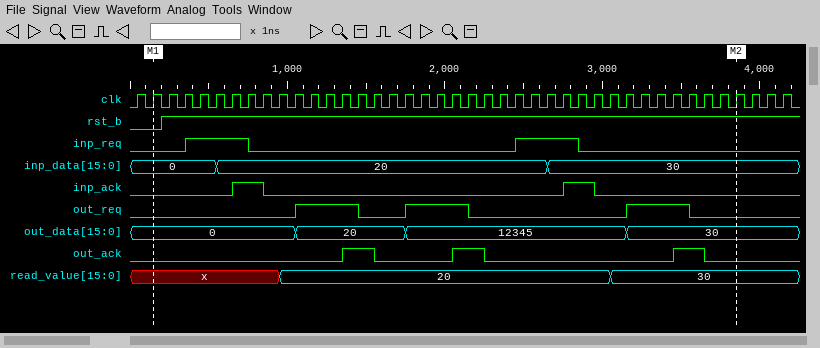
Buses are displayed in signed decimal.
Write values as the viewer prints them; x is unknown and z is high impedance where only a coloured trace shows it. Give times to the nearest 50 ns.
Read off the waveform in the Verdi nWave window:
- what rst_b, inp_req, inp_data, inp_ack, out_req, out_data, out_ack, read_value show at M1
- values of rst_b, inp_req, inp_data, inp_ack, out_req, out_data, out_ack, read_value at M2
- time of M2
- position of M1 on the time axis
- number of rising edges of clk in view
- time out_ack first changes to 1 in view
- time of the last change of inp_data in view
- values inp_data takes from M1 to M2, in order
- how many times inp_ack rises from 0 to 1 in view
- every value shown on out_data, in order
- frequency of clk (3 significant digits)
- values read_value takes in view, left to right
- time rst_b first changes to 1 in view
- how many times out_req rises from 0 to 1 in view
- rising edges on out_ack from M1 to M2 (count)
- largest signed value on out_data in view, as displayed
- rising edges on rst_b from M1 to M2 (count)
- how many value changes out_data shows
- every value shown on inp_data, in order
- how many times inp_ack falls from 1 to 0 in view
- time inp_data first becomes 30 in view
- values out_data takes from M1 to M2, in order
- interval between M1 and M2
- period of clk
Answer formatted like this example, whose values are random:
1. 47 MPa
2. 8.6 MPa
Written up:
1. rst_b=0, inp_req=0, inp_data=0, inp_ack=0, out_req=0, out_data=0, out_ack=0, read_value=x
2. rst_b=1, inp_req=0, inp_data=30, inp_ack=0, out_req=0, out_data=30, out_ack=0, read_value=30
3. 3850 ns
4. 150 ns
5. 42
6. 1350 ns
7. 2650 ns
8. 0, 20, 30
9. 2
10. 0, 20, 12345, 30
11. 10.0 MHz
12. x, 20, 30
13. 200 ns
14. 3
15. 3
16. 12345
17. 1
18. 3
19. 0, 20, 30
20. 2
21. 2650 ns
22. 0, 20, 12345, 30
23. 3700 ns
24. 100 ns
